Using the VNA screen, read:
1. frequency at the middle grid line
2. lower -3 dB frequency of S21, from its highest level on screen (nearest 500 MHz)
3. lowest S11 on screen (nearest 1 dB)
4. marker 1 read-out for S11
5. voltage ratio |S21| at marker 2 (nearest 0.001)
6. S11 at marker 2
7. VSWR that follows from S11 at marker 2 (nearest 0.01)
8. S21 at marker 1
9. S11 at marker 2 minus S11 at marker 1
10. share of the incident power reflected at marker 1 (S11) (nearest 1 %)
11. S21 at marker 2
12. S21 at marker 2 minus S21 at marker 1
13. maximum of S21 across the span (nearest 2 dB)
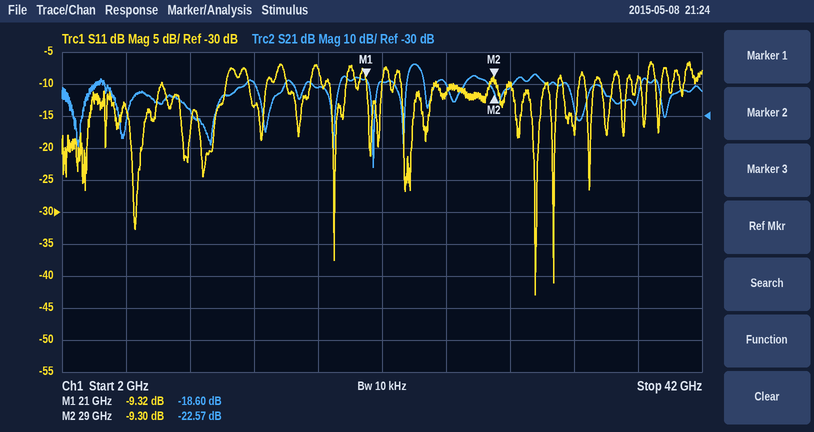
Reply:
22 GHz
23.5 GHz
-43 dB
-9.32 dB
0.074
-9.30 dB
2.04
-18.60 dB
0.02 dB
12 %
-22.57 dB
-3.97 dB
-14 dB
